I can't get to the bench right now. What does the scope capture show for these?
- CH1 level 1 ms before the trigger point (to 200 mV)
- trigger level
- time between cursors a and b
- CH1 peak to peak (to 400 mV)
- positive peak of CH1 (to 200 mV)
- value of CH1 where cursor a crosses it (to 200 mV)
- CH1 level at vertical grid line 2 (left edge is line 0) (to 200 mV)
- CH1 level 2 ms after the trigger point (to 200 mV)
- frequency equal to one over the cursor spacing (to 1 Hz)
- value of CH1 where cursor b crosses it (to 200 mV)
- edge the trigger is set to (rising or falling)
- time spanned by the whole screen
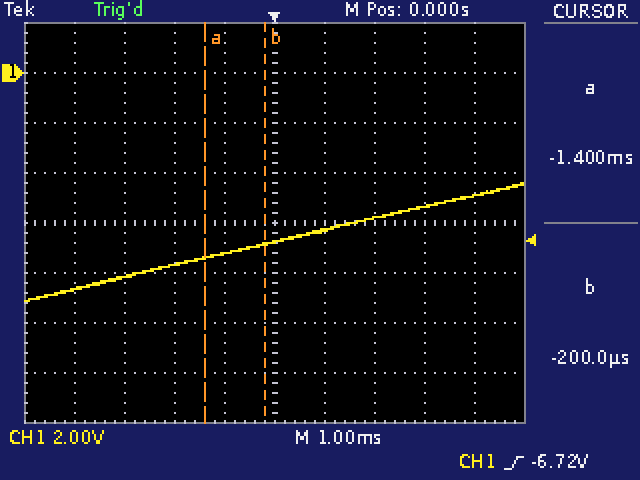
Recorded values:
-7.2 V
-6.72 V
1.2 ms
4.8 V
-4.4 V
-7.4 V
-8.2 V
-5.8 V
833 Hz
-6.8 V
rising
10 ms
